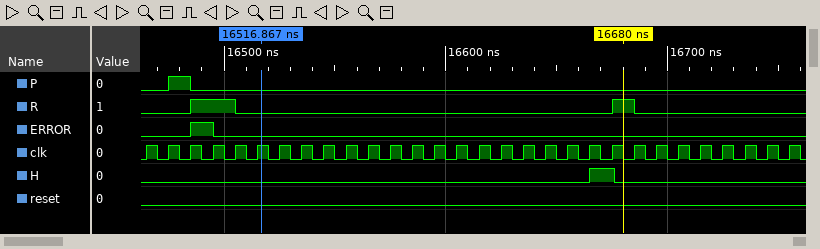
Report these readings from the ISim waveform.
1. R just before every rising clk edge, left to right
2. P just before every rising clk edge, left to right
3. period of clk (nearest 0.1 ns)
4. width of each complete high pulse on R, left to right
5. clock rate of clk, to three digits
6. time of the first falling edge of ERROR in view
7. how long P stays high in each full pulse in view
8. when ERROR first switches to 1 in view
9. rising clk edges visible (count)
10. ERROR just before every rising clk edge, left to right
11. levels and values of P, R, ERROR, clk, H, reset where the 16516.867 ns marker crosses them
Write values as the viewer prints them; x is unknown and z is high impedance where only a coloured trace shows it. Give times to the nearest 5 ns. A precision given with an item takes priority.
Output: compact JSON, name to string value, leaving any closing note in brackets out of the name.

{"R just before every rising clk edge, left to right": "0 0 0 1 1 0 0 0 0 0 0 0 0 0 0 0 0 0 0 0 0 0 1 0 0 0 0 0 0 0", "P just before every rising clk edge, left to right": "0 0 1 0 0 0 0 0 0 0 0 0 0 0 0 0 0 0 0 0 0 0 0 0 0 0 0 0 0 0", "period of clk": "10 ns", "width of each complete high pulse on R, left to right": "20 ns, 10 ns", "clock rate of clk, to three digits": "100 MHz", "time of the first falling edge of ERROR in view": "16495 ns", "how long P stays high in each full pulse in view": "10 ns", "when ERROR first switches to 1 in view": "16485 ns", "rising clk edges visible": "30", "ERROR just before every rising clk edge, left to right": "0 0 0 1 0 0 0 0 0 0 0 0 0 0 0 0 0 0 0 0 0 0 0 0 0 0 0 0 0 0", "levels and values of P, R, ERROR, clk, H, reset where the 16516.867 ns marker crosses them": "P=0, R=0, ERROR=0, clk=1, H=0, reset=0"}
